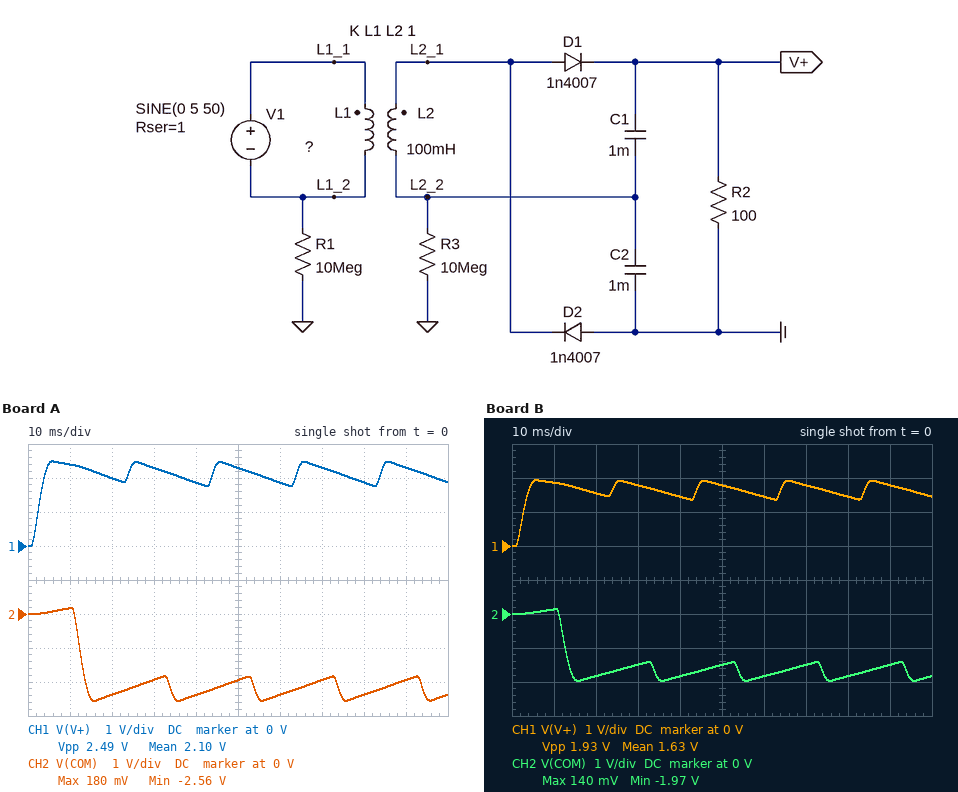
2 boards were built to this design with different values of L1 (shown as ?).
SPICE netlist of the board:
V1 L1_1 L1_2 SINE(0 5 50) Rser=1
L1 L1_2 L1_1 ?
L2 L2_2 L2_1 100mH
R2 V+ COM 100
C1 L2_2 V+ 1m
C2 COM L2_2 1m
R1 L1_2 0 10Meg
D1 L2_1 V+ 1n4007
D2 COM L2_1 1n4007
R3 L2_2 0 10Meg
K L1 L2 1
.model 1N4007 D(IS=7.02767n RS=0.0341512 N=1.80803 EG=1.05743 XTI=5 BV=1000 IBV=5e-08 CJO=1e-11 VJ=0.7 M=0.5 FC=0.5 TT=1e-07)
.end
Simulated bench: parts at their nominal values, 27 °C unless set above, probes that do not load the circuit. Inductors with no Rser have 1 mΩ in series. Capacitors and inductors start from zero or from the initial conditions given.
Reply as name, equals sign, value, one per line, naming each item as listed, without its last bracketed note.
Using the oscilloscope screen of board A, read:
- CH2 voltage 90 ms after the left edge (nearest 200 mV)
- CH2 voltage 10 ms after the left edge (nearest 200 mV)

CH2 voltage 90 ms after the left edge = -2.0 V
CH2 voltage 10 ms after the left edge = 200 mV
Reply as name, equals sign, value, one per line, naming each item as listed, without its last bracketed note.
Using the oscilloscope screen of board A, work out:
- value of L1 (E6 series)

value of L1 = 220 mH
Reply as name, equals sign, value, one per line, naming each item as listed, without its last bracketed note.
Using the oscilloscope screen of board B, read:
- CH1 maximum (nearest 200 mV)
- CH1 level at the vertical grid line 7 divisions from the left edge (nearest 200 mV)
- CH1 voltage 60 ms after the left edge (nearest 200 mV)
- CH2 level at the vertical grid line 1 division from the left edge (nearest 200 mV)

CH1 maximum = 2.0 V
CH1 level at the vertical grid line 7 divisions from the left edge = 1.8 V
CH1 voltage 60 ms after the left edge = 1.4 V
CH2 level at the vertical grid line 1 division from the left edge = 200 mV
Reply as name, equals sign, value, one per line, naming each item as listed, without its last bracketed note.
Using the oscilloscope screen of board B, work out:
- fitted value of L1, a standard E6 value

fitted value of L1, a standard E6 value = 330 mH
